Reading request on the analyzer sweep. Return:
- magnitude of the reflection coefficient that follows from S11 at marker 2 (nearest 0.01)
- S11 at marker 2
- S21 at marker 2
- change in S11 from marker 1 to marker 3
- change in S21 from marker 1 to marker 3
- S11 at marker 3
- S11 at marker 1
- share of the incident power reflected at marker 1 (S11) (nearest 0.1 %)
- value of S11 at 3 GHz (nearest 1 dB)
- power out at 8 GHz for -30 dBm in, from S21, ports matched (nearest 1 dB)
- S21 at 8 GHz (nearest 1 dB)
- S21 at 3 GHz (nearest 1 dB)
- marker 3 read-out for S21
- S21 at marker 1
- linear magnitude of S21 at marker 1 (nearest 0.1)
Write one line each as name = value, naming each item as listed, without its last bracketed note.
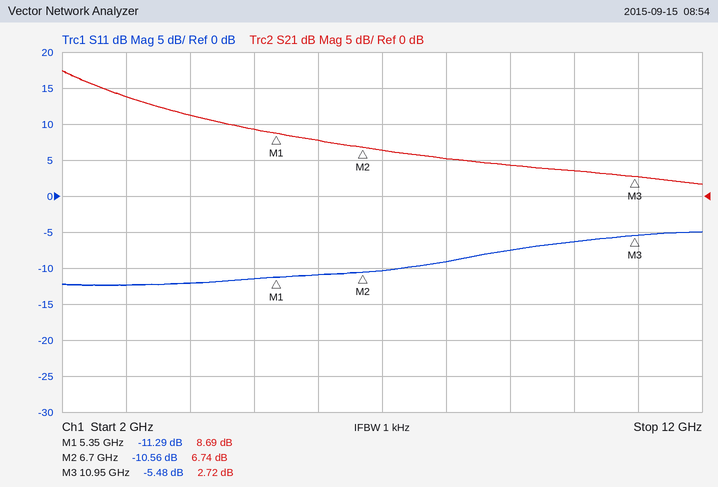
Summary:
magnitude of the reflection coefficient that follows from S11 at marker 2 = 0.30
S11 at marker 2 = -10.56 dB
S21 at marker 2 = 6.74 dB
change in S11 from marker 1 to marker 3 = 5.81 dB
change in S21 from marker 1 to marker 3 = -5.97 dB
S11 at marker 3 = -5.48 dB
S11 at marker 1 = -11.29 dB
share of the incident power reflected at marker 1 (S11) = 7.4 %
value of S11 at 3 GHz = -12 dB
power out at 8 GHz for -30 dBm in, from S21, ports matched = -25 dBm
S21 at 8 GHz = 5 dB
S21 at 3 GHz = 14 dB
marker 3 read-out for S21 = 2.72 dB
S21 at marker 1 = 8.69 dB
linear magnitude of S21 at marker 1 = 2.7
